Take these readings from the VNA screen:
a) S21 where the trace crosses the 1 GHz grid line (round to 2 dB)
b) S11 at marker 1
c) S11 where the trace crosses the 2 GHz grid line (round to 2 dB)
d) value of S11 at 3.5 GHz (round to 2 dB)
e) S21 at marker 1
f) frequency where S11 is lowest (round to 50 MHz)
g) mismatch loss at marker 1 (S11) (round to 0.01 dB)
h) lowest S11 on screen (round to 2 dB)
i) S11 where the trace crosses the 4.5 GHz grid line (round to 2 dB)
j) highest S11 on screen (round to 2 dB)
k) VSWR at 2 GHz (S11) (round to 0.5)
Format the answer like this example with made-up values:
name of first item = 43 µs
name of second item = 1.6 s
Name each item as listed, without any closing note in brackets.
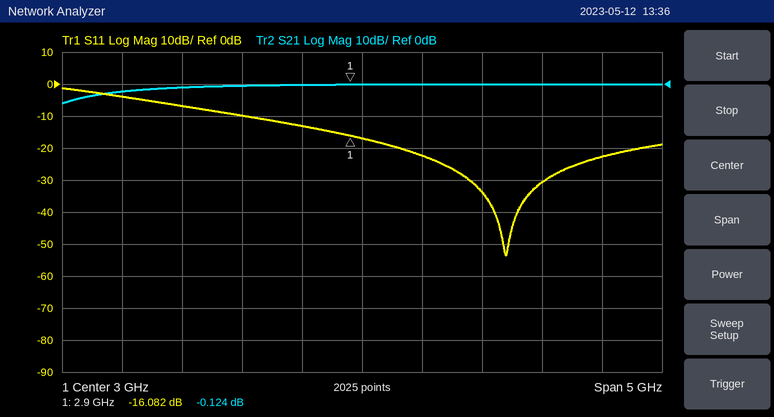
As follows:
S21 where the trace crosses the 1 GHz grid line = -2 dB
S11 at marker 1 = -16.082 dB
S11 where the trace crosses the 2 GHz grid line = -10 dB
value of S11 at 3.5 GHz = -22 dB
S21 at marker 1 = -0.124 dB
frequency where S11 is lowest = 4.20 GHz
mismatch loss at marker 1 (S11) = 0.11 dB
lowest S11 on screen = -54 dB
S11 where the trace crosses the 4.5 GHz grid line = -30 dB
highest S11 on screen = -2 dB
VSWR at 2 GHz (S11) = 2.0
